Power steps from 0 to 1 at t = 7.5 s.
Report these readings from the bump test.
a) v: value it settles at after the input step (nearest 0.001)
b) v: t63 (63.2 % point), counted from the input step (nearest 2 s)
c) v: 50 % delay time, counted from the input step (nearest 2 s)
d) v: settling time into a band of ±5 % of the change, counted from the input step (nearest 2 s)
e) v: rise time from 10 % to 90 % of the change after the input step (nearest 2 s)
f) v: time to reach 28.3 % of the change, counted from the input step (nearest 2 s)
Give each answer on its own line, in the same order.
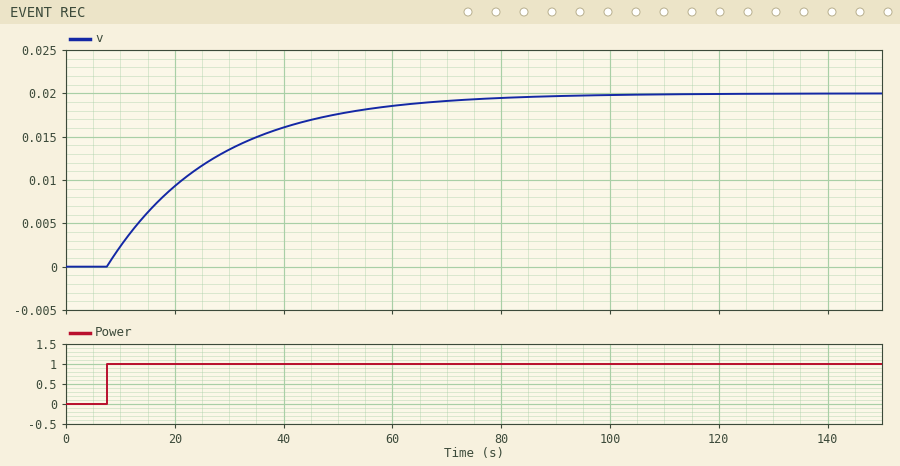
0.020
20 s
14 s
60 s
44 s
6 s
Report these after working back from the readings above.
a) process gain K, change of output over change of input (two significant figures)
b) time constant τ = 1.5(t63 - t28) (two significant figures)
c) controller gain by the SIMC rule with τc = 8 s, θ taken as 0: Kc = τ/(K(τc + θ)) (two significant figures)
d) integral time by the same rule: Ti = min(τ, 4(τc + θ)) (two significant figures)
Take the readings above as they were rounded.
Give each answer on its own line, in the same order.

0.020
21 s
130
21 s
